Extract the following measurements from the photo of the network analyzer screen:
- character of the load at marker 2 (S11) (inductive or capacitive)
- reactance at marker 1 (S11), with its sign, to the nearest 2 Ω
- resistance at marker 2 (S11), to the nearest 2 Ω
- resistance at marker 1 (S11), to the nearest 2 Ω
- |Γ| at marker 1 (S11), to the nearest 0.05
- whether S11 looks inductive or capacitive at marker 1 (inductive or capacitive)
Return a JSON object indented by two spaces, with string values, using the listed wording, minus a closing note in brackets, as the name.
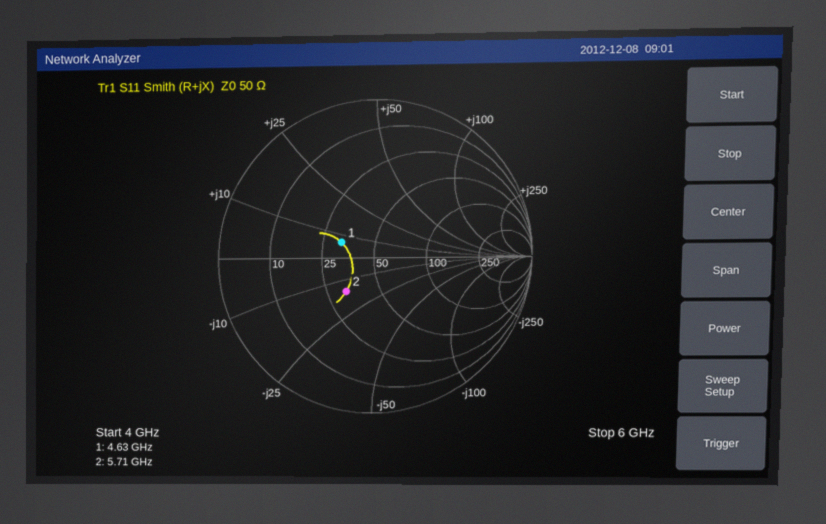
{
  "character of the load at marker 2 (S11)": "capacitive",
  "reactance at marker 1 (S11), with its sign, to the nearest 2 Ω": "+6 Ω",
  "resistance at marker 2 (S11), to the nearest 2 Ω": "32 Ω",
  "resistance at marker 1 (S11), to the nearest 2 Ω": "32 Ω",
  "|Γ| at marker 1 (S11), to the nearest 0.05": "0.25",
  "whether S11 looks inductive or capacitive at marker 1": "inductive"
}
